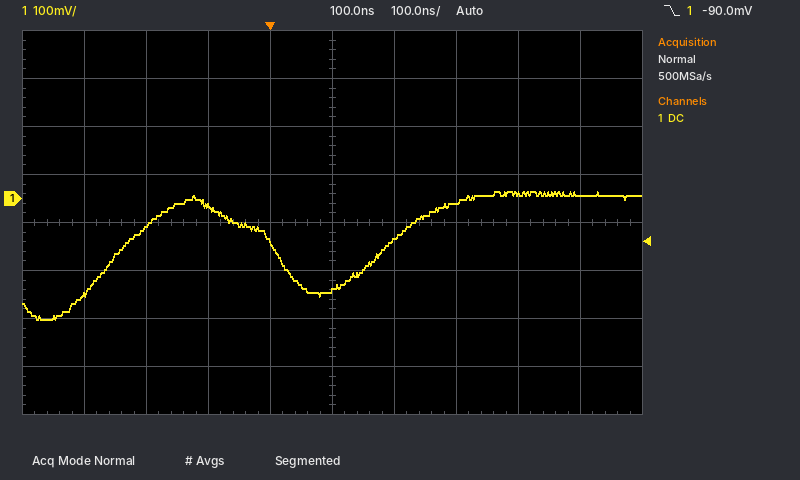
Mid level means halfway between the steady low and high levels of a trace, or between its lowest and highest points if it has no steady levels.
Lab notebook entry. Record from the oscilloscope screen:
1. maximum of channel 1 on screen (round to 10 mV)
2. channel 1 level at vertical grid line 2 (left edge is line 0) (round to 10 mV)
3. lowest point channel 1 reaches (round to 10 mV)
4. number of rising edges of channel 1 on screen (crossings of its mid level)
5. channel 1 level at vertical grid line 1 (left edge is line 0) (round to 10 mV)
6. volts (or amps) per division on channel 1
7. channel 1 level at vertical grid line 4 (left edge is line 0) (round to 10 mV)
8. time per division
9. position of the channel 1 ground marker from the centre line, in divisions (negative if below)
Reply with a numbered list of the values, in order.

1. 10 mV
2. -60 mV
3. -250 mV
4. 2
5. -200 mV
6. 100 mV
7. -90 mV
8. 100 ns
9. +0.5 div
